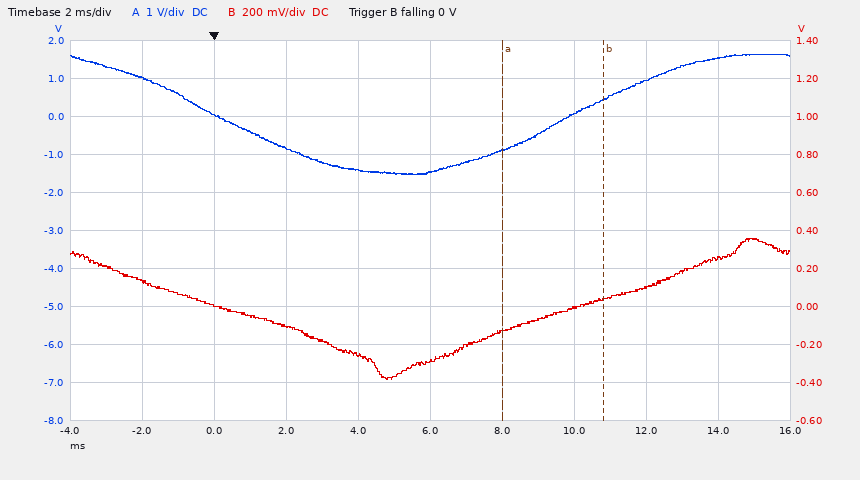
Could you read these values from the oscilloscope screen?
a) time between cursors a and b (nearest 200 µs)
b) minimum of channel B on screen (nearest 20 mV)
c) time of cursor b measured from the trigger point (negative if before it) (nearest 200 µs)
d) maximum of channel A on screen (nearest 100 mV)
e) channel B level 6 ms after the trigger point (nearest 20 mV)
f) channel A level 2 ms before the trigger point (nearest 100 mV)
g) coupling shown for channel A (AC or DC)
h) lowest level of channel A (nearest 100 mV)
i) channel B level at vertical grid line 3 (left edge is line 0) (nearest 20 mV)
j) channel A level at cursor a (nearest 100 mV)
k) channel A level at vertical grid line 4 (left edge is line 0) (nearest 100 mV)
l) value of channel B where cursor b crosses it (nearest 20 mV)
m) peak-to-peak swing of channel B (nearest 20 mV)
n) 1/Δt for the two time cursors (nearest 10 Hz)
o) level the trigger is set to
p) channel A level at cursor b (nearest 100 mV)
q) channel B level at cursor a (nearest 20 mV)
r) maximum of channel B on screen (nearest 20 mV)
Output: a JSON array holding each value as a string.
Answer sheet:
["2.8 ms", "-380 mV", "+10.8 ms", "1.6 V", "-280 mV", "1.0 V", "DC", "-1.5 V", "-100 mV", "-900 mV", "-1.4 V", "40 mV", "740 mV", "360 Hz", "0 V", "400 mV", "-140 mV", "360 mV"]
